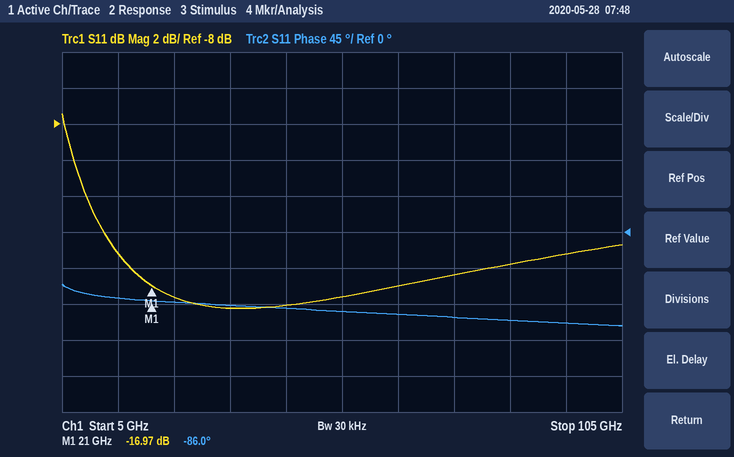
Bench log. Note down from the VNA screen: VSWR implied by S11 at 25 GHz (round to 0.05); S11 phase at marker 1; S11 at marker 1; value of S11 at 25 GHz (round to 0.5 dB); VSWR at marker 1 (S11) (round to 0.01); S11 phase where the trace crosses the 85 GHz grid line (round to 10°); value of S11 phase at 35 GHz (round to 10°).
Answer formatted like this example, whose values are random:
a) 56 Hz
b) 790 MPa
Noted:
a) 1.30
b) -86.0°
c) -16.97 dB
d) -17.5 dB
e) 1.33
f) -110°
g) -90°
